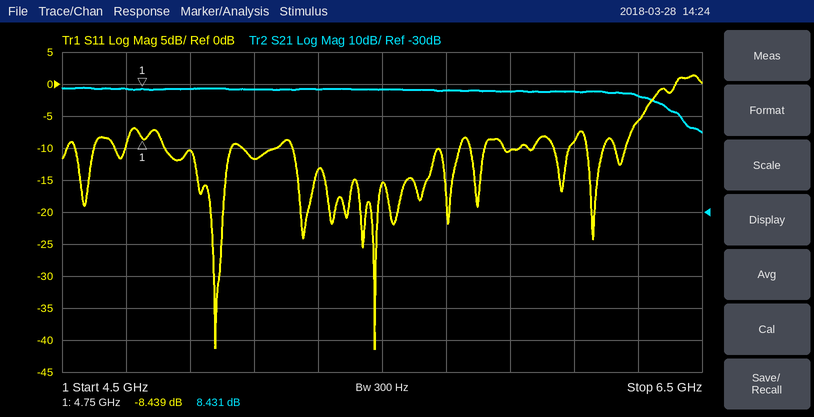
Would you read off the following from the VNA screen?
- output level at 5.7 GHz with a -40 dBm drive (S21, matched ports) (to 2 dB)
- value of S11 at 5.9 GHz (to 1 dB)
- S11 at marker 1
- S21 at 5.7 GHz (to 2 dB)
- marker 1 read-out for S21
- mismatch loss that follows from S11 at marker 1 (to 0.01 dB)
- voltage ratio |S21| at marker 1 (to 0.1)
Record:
-32 dBm
-10 dB
-8.439 dB
8 dB
8.431 dB
0.67 dB
2.6
